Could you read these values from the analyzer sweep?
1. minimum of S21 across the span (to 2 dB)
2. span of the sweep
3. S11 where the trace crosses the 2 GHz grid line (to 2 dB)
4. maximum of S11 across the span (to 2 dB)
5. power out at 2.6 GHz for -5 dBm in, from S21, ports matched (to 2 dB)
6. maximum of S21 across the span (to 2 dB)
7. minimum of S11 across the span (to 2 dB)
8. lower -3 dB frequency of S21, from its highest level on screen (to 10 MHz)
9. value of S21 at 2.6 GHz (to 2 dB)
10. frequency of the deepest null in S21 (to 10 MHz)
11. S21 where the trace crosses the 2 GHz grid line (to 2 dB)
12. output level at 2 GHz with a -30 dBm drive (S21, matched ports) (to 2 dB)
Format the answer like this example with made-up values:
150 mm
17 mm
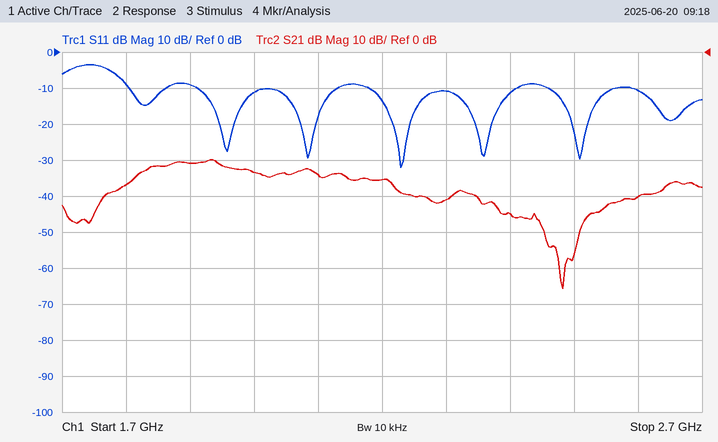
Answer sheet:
-66 dB
1 GHz
-12 dB
-4 dB
-46 dBm
-30 dB
-32 dB
1.83 GHz
-40 dB
2.48 GHz
-34 dB
-64 dBm
